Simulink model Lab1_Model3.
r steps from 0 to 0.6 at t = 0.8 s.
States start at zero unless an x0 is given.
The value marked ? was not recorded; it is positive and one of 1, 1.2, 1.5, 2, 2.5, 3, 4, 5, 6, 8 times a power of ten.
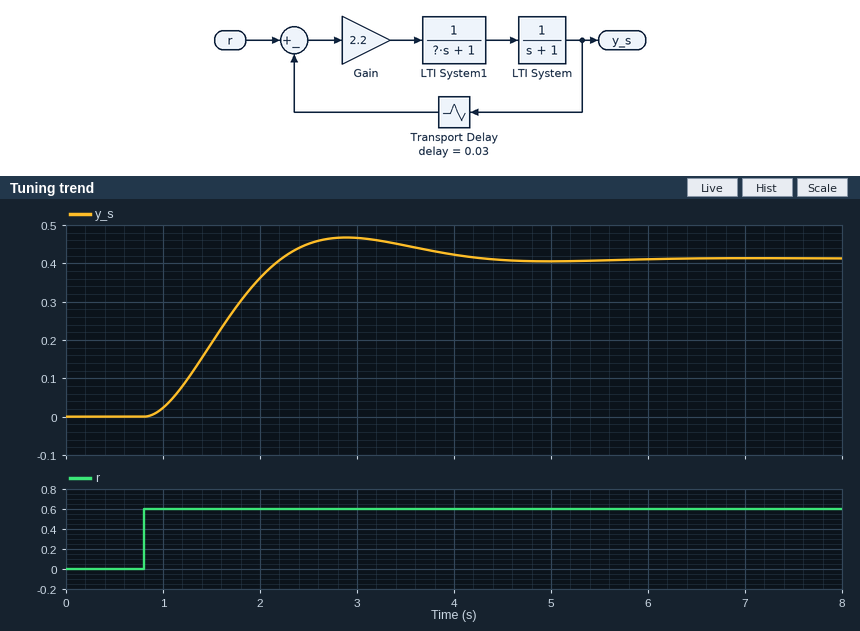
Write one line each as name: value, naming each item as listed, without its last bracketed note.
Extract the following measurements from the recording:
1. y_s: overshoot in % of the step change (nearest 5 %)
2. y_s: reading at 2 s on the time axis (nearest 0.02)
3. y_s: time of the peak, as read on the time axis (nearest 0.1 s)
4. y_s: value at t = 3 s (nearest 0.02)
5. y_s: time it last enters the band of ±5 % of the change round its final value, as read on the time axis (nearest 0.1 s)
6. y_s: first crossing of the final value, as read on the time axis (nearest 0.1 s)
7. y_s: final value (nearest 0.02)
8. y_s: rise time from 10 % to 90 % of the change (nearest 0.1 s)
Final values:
y_s: overshoot in % of the step change: 15 %
y_s: reading at 2 s on the time axis: 0.36
y_s: time of the peak, as read on the time axis: 2.9 s
y_s: value at t = 3 s: 0.46
y_s: time it last enters the band of ±5 % of the change round its final value, as read on the time axis: 3.8 s
y_s: first crossing of the final value, as read on the time axis: 2.2 s
y_s: final value: 0.42
y_s: rise time from 10 % to 90 % of the change: 1.0 s
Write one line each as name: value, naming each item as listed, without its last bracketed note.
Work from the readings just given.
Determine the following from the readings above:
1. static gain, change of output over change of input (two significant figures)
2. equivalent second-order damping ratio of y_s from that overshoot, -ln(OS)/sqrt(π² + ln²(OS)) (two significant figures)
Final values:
static gain, change of output over change of input: 0.70
equivalent second-order damping ratio of y_s from that overshoot, -ln(OS)/sqrt(π² + ln²(OS)): 0.52
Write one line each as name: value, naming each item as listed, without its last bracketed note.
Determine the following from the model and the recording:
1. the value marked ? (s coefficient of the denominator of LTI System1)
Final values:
the value marked ?: 1
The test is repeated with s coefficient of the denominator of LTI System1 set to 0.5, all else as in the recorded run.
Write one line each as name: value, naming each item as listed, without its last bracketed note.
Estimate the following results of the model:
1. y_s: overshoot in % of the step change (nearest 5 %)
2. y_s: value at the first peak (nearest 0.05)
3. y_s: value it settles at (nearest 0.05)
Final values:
y_s: overshoot in % of the step change: 10 %
y_s: value at the first peak: 0.45
y_s: value it settles at: 0.40
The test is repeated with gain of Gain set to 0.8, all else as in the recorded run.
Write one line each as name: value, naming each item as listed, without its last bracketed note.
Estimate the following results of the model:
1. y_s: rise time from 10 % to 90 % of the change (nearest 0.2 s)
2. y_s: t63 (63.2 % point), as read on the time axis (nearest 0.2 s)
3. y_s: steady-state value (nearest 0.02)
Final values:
y_s: rise time from 10 % to 90 % of the change: 1.6 s
y_s: t63 (63.2 % point), as read on the time axis: 2.2 s
y_s: steady-state value: 0.26
